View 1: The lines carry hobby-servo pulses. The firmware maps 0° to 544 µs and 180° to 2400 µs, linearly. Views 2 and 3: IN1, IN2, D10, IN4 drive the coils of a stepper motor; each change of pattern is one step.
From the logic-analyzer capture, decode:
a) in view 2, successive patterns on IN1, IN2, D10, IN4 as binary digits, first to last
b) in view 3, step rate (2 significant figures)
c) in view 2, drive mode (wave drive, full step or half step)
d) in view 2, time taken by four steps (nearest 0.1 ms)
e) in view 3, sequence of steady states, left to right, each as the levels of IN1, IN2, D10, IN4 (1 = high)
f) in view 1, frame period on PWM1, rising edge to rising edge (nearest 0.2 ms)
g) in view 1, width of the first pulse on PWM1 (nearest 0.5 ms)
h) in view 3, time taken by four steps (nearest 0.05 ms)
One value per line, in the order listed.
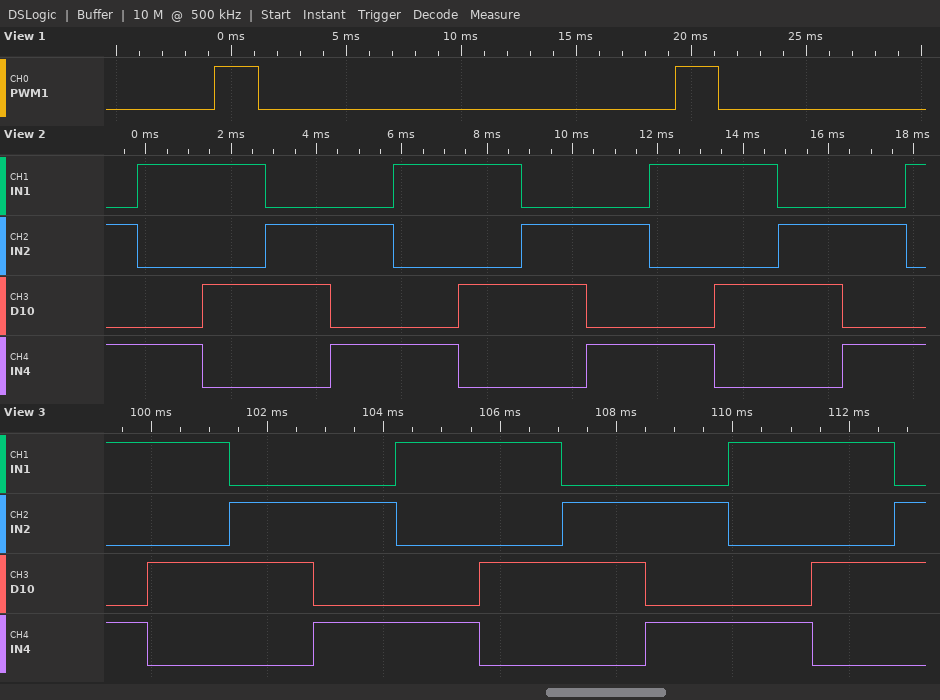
0101 1001 1010 0110 0101 1001 1010 0110 0101 1001 1010 0110 0101 1001
700 steps/s
full step
6.0 ms
1001 1010 0110 0101 1001 1010 0110 0101 1001 1010 0110
20.0 ms
2.0 ms
5.70 ms
